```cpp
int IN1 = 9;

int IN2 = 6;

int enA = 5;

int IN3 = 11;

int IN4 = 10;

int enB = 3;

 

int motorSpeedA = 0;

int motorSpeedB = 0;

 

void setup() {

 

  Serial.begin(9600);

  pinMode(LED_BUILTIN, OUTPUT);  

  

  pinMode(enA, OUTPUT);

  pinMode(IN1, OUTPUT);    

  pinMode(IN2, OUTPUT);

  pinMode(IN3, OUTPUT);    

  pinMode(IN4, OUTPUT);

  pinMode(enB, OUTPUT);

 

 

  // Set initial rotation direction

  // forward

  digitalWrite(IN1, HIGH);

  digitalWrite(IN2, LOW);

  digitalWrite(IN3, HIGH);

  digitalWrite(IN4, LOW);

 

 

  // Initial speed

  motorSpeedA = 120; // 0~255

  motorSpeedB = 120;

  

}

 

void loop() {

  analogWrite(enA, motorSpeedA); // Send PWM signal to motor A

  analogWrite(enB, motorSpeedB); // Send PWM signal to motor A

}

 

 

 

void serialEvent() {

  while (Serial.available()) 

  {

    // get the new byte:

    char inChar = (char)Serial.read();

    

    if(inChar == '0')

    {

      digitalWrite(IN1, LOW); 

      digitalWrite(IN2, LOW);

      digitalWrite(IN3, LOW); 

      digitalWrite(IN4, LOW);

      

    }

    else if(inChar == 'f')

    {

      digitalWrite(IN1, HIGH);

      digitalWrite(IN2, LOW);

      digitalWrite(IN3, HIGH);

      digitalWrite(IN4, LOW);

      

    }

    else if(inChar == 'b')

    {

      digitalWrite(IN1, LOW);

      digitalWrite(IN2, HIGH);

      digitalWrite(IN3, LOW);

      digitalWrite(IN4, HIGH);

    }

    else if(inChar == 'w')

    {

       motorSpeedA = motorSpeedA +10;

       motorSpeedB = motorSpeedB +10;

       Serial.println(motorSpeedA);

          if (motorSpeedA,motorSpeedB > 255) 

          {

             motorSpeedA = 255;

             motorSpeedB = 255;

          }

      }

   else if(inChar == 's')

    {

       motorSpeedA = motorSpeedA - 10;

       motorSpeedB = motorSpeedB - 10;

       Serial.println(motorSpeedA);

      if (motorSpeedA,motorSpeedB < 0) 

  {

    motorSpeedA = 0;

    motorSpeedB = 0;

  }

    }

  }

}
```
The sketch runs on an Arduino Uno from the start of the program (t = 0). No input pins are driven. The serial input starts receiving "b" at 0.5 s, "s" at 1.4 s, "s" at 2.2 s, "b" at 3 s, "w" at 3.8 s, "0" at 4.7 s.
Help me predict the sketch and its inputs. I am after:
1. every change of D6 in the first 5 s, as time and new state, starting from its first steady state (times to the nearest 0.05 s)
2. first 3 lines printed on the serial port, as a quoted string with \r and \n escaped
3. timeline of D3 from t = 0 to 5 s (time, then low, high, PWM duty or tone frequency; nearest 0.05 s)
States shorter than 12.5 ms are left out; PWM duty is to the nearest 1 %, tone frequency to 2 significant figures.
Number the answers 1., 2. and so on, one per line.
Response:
1. 0 s low; 0.5 s high; 4.7 s low
2. "110\r\n100\r\n110\r\n"
3. 0 s PWM 47 %; 1.4 s PWM 43 %; 2.2 s PWM 39 %; 3.8 s PWM 43 %
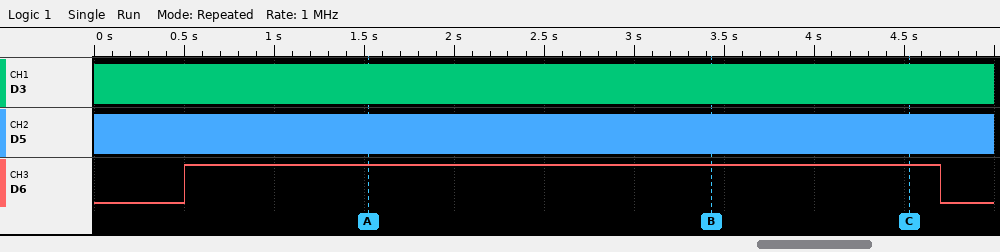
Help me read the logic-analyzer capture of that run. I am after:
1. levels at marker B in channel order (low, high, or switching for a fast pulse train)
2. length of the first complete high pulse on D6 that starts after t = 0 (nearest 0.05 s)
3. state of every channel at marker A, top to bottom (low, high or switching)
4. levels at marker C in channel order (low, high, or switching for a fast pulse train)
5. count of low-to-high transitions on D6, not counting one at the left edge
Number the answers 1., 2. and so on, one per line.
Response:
1. D3 switching, D5 switching, D6 high
2. 4.20 s
3. D3 switching, D5 switching, D6 high
4. D3 switching, D5 switching, D6 high
5. 1
